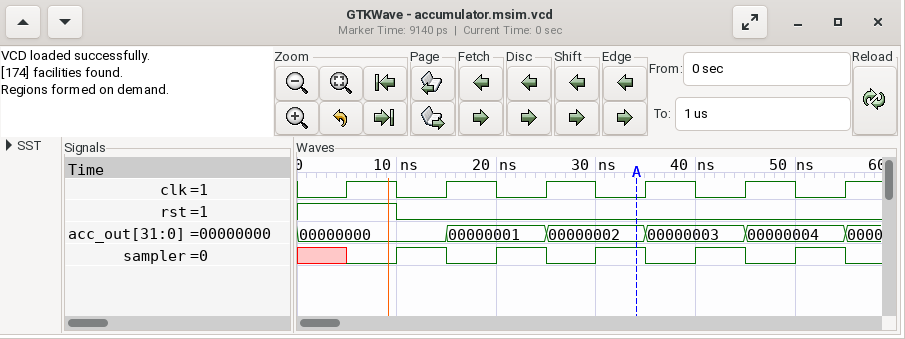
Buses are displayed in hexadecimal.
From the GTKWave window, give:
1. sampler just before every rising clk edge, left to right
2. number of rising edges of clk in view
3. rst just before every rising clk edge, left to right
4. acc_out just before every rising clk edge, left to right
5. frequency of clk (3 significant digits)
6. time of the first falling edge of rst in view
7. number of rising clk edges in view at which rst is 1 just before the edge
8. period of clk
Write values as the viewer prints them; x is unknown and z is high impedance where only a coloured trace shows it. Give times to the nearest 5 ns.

x 1 1 1 1 1
6
1 0 0 0 0 0
00000000, 00000000, 00000001, 00000002, 00000003, 00000004
100 MHz
10 ns
1
10 ns
